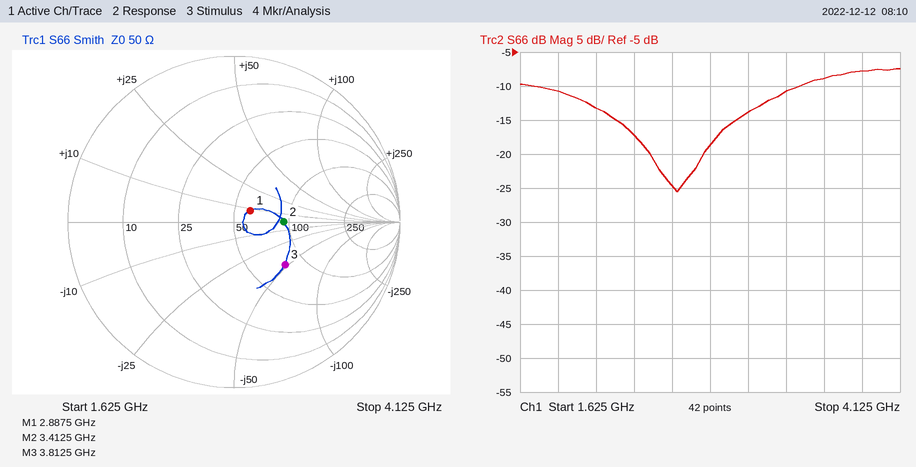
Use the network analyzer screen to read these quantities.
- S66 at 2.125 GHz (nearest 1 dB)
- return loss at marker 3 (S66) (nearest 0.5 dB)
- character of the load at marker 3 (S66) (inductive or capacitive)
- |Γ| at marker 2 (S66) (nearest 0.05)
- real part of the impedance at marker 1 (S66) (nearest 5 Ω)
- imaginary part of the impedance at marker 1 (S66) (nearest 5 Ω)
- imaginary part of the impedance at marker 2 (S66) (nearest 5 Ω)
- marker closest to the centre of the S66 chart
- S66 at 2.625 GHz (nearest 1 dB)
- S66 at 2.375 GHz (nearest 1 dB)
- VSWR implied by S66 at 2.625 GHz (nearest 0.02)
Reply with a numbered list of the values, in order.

1. -13 dB
2. 8.0 dB
3. capacitive
4. 0.30
5. 60 Ω
6. +10 Ω
7. 0 Ω
8. marker 1
9. -25 dB
10. -17 dB
11. 1.12
